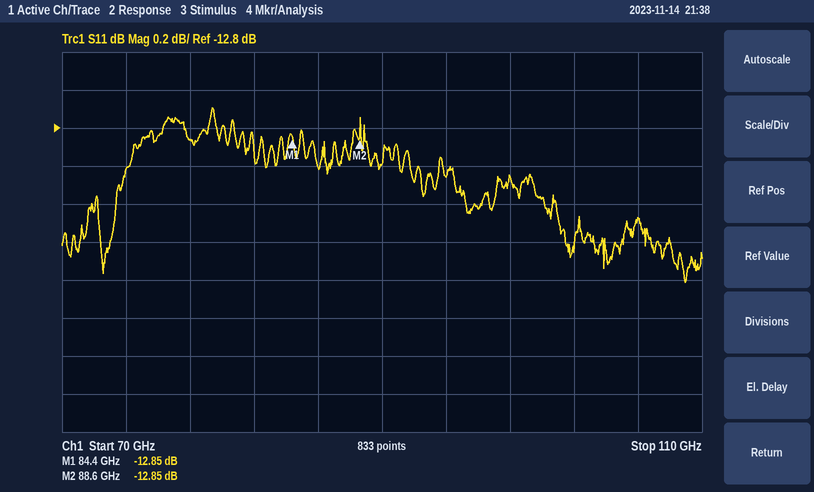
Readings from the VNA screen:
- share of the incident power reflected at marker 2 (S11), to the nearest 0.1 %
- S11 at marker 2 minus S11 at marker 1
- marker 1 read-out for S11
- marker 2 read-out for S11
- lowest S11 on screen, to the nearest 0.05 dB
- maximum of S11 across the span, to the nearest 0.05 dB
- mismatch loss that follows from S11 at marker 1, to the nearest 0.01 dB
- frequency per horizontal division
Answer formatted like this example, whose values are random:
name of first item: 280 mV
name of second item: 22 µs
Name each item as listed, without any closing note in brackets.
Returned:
share of the incident power reflected at marker 2 (S11), to the nearest 0.1 %: 5.2 %
S11 at marker 2 minus S11 at marker 1: 0.00 dB
marker 1 read-out for S11: -12.85 dB
marker 2 read-out for S11: -12.85 dB
lowest S11 on screen, to the nearest 0.05 dB: -13.60 dB
maximum of S11 across the span, to the nearest 0.05 dB: -12.70 dB
mismatch loss that follows from S11 at marker 1, to the nearest 0.01 dB: 0.23 dB
frequency per horizontal division: 4 GHz
